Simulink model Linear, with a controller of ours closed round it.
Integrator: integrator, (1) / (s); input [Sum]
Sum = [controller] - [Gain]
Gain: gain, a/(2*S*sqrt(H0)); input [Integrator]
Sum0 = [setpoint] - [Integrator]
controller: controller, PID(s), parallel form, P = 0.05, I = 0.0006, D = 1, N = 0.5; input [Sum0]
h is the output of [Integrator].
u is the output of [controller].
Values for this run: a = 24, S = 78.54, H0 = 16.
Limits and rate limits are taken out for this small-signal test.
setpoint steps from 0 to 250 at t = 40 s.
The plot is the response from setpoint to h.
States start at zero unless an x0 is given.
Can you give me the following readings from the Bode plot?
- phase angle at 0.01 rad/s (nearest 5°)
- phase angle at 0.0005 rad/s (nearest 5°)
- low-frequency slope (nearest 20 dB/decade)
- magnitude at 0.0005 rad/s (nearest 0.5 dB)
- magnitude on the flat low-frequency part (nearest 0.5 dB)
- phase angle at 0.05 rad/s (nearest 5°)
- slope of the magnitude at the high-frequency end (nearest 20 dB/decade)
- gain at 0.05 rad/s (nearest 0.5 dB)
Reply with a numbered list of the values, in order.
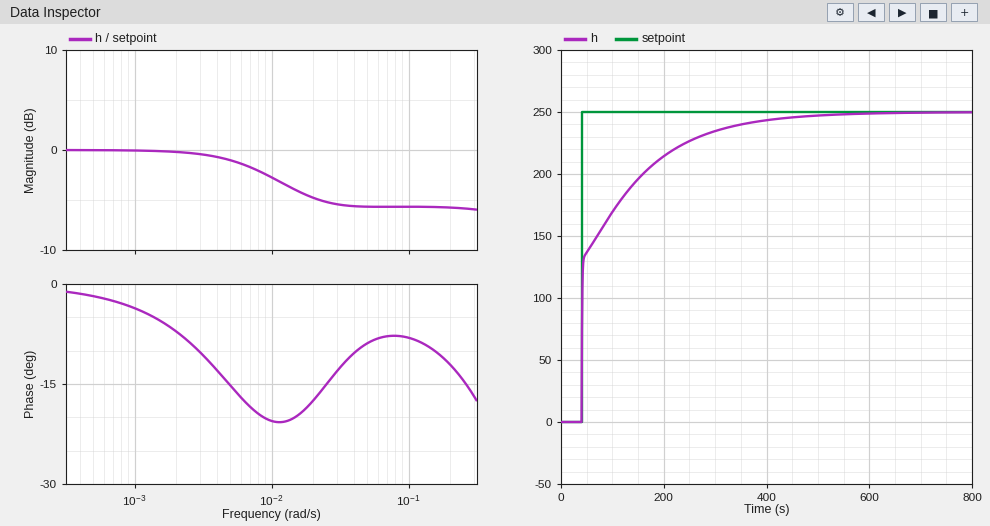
1. -20°
2. 0°
3. 0 dB/decade
4. 0.0 dB
5. 0.0 dB
6. -10°
7. 0 dB/decade
8. -5.5 dB
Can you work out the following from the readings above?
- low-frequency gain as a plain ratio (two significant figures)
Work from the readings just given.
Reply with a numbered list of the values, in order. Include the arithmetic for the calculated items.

1. 10^(0 / 20) = 1.0
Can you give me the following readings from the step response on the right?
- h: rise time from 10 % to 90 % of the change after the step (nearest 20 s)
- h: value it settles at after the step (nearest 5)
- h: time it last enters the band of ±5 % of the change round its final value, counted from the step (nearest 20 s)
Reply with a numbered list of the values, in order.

1. 200 s
2. 250
3. 280 s
